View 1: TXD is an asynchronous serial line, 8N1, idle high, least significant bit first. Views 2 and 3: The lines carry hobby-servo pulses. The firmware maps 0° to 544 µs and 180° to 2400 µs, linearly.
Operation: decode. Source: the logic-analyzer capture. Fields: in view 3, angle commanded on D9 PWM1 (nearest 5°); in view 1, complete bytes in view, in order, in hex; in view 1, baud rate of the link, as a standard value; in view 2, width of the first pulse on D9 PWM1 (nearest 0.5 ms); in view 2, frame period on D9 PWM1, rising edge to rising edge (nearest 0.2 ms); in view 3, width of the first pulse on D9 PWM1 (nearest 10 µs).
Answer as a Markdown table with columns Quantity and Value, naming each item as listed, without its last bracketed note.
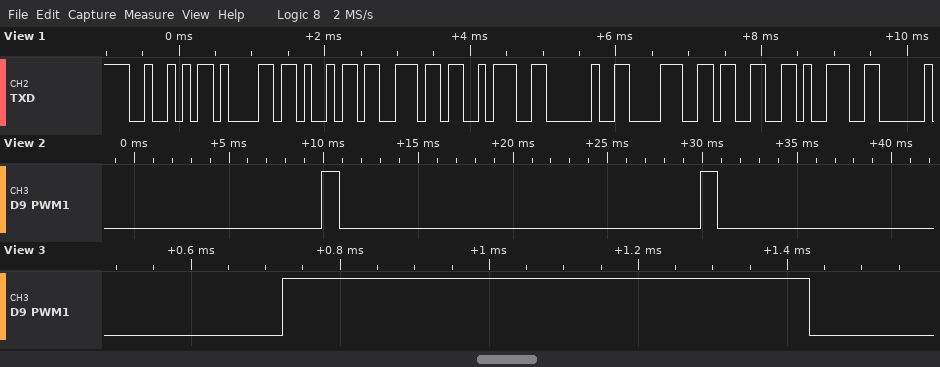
| Quantity | Value |
|---|---|
| in view 3, angle commanded on D9 PWM1 | 15° |
| in view 1, complete bytes in view, in order, in hex | 52 61 69 6E 3A 20 38 33 39 |
| in view 1, baud rate of the link, as a standard value | 9600 baud |
| in view 2, width of the first pulse on D9 PWM1 | 1.0 ms |
| in view 2, frame period on D9 PWM1, rising edge to rising edge | 20.0 ms |
| in view 3, width of the first pulse on D9 PWM1 | 710 µs |
